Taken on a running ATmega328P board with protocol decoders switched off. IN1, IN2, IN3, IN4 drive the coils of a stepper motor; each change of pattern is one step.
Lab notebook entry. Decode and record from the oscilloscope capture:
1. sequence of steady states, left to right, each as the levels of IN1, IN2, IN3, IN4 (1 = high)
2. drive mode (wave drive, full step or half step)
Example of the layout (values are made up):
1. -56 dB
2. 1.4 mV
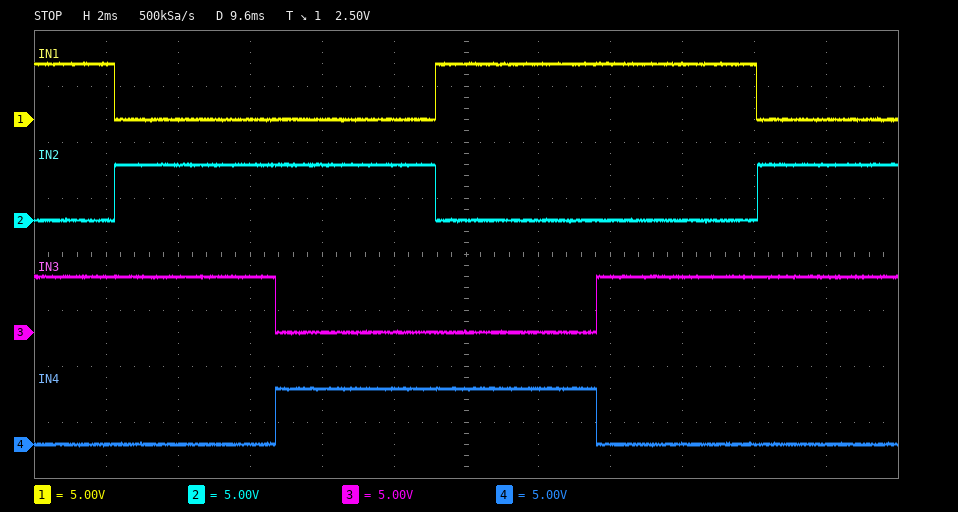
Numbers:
1. 1010 0110 0101 1001 1010 0110
2. full step
